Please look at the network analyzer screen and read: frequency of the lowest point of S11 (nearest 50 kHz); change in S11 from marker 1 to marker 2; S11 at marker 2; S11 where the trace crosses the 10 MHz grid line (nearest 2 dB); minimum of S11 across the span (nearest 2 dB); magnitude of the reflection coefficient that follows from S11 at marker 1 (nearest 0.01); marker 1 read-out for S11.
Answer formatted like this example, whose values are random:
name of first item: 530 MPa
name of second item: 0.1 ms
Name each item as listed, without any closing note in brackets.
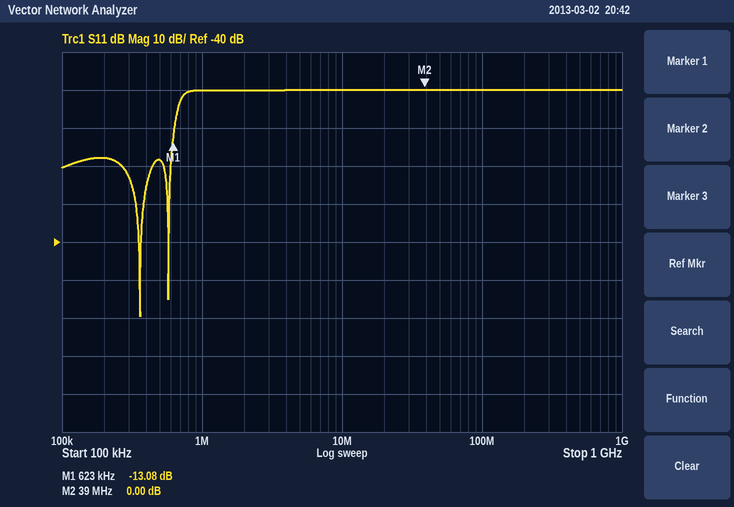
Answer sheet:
frequency of the lowest point of S11: 350 kHz
change in S11 from marker 1 to marker 2: 13.08 dB
S11 at marker 2: 0.00 dB
S11 where the trace crosses the 10 MHz grid line: 0 dB
minimum of S11 across the span: -60 dB
magnitude of the reflection coefficient that follows from S11 at marker 1: 0.22
marker 1 read-out for S11: -13.08 dB
